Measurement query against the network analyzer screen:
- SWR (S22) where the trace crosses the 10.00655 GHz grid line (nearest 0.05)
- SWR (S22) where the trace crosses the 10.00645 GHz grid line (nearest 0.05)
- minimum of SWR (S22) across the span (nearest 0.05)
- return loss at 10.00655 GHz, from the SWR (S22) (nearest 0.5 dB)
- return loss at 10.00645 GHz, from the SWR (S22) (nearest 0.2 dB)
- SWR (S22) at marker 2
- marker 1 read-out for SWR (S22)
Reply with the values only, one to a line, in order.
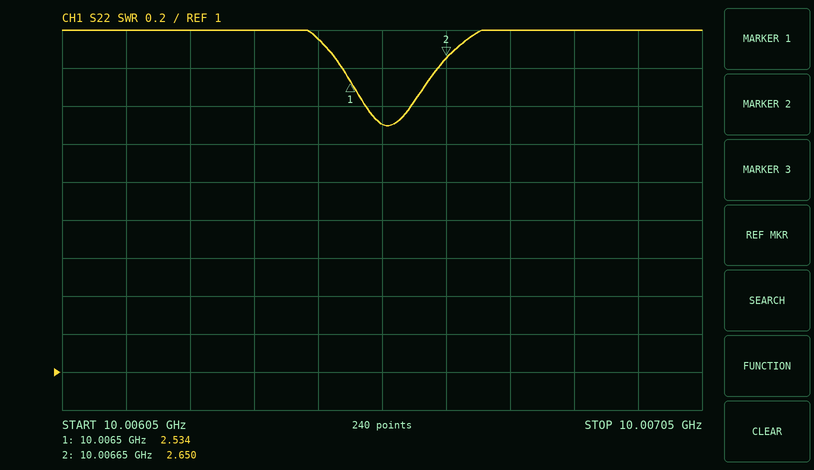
2.30
2.75
2.30
8.0 dB
6.6 dB
2.650
2.534
